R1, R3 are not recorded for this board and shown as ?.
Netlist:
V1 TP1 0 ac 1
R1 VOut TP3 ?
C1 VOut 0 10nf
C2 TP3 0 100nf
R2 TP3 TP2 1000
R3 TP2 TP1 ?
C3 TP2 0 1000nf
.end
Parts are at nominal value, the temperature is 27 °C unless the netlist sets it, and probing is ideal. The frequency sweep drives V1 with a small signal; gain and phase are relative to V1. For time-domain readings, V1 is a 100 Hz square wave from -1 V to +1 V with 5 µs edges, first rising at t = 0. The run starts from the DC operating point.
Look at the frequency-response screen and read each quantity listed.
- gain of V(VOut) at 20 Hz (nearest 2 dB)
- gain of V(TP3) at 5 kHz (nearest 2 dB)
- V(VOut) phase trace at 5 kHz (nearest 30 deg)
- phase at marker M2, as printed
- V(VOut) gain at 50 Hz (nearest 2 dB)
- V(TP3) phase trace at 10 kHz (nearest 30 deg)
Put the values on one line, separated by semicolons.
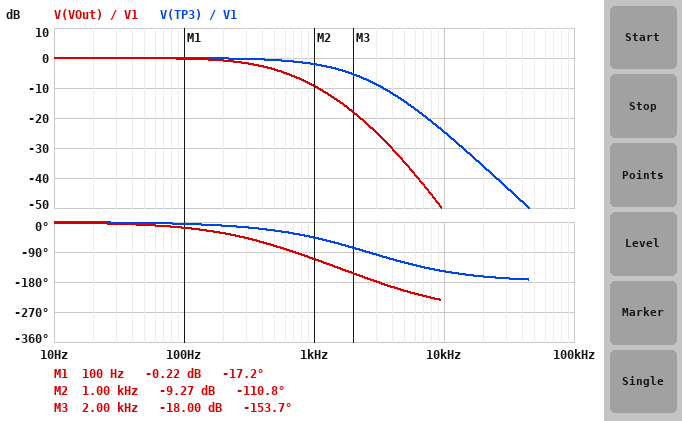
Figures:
0 dB; -14 dB; -210 deg; -110.8 deg; 0 dB; -150 deg
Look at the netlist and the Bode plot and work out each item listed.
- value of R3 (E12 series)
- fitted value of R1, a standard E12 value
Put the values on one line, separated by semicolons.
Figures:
39 Ω; 33 kΩ
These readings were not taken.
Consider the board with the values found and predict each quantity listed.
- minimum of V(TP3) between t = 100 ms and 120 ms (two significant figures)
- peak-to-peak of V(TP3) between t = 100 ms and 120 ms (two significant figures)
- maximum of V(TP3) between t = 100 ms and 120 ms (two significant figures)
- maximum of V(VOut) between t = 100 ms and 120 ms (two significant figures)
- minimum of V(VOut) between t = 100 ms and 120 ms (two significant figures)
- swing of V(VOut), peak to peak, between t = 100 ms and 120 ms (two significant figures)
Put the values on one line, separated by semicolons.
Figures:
-1.0 V; 2.0 V; 1.0 V; 1.0 V; -1.0 V; 2.0 V
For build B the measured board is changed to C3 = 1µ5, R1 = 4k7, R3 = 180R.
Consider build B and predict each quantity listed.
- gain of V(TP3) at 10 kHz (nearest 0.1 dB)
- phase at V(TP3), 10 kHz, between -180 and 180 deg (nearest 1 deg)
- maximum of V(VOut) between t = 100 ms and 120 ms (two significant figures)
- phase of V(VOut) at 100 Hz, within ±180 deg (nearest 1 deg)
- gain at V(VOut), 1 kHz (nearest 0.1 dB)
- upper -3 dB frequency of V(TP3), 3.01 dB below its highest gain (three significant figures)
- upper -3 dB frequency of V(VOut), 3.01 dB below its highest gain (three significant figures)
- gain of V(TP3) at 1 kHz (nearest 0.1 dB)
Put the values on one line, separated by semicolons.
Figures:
-40.8 dB; -165 deg; 1.0 V; -16 deg; -8.5 dB; 480 Hz; 471 Hz; -8.1 dB
